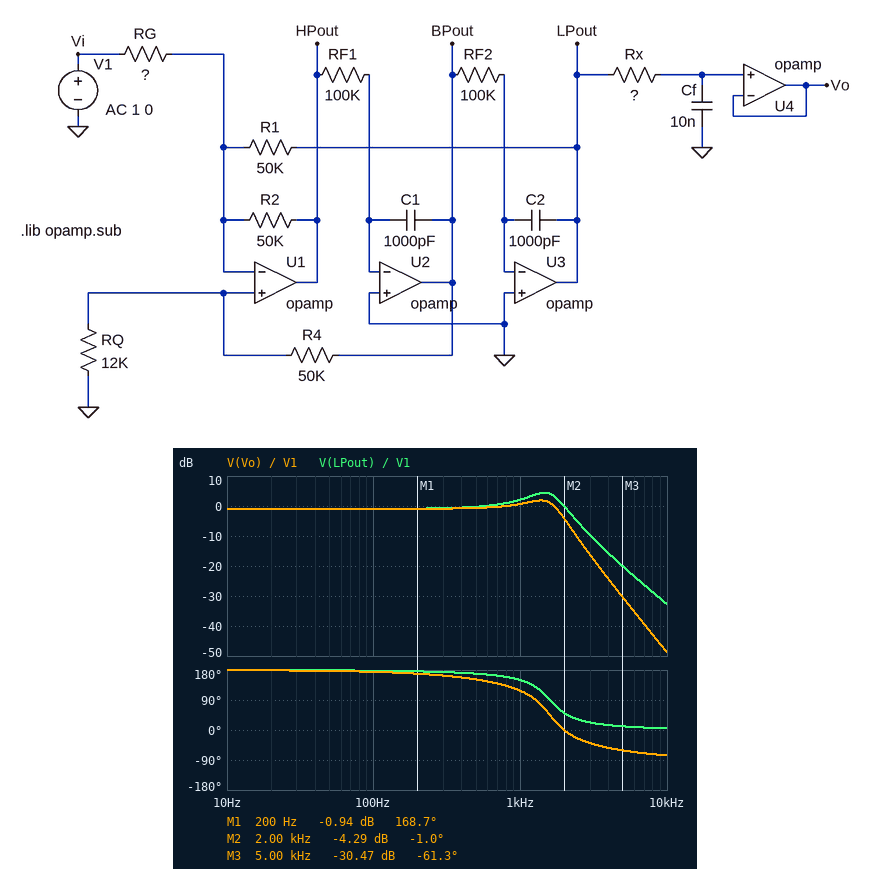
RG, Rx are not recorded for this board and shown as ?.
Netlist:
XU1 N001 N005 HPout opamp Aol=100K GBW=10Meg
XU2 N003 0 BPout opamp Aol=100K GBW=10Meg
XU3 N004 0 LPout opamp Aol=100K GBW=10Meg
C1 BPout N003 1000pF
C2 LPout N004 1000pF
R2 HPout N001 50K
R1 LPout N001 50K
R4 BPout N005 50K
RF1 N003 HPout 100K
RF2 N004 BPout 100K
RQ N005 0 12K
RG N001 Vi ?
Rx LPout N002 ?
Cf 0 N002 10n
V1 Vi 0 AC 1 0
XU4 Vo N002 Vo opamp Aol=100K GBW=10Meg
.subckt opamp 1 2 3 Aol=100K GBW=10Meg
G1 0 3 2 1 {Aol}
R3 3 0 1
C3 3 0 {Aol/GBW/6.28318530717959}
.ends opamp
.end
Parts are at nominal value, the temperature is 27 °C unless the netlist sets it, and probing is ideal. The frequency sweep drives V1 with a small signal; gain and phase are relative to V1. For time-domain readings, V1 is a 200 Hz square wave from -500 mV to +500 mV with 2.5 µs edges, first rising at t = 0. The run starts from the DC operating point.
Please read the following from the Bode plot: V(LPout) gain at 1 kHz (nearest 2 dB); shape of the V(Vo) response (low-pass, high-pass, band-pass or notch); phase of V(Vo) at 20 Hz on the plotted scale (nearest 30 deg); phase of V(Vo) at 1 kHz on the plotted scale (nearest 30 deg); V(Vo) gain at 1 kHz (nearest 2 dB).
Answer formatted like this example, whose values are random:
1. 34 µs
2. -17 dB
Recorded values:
1. 2 dB
2. low-pass
3. 180 deg
4. 120 deg
5. 0 dB
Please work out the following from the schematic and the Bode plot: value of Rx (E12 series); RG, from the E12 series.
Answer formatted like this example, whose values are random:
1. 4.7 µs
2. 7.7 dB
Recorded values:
1. 10 kΩ
2. 56 kΩ
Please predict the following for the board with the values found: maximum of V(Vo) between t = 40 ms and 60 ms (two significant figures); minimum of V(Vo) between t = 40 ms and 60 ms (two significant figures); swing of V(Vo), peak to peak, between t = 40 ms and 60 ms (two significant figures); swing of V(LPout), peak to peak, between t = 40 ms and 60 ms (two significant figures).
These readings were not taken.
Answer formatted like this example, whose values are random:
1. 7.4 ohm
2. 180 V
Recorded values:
1. 670 mV
2. -670 mV
3. 1.3 V
4. 1.6 V
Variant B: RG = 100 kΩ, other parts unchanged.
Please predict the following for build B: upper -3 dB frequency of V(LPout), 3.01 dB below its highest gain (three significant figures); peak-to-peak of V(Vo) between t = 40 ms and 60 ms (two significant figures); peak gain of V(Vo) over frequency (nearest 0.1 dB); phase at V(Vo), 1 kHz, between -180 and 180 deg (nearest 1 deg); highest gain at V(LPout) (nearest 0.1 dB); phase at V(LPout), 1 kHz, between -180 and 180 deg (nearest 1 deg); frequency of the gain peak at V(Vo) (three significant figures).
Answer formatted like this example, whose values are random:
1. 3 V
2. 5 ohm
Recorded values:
1. 1.85 kHz
2. 790 mV
3. -2.1 dB
4. 121 deg
5. 0.6 dB
6. 153 deg
7. 1.44 kHz
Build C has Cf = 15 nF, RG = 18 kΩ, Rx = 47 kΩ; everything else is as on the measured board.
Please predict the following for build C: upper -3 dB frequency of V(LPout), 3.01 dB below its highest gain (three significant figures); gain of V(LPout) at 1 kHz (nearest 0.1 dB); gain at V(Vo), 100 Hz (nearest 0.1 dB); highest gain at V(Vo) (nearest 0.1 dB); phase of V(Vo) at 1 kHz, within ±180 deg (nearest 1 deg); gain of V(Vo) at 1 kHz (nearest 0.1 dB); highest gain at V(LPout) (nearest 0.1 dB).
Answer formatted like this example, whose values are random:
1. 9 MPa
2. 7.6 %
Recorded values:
1. 1.88 kHz
2. 10.4 dB
3. 8.1 dB
4. 8.9 dB
5. 59 deg
6. -2.7 dB
7. 10.6 dB
